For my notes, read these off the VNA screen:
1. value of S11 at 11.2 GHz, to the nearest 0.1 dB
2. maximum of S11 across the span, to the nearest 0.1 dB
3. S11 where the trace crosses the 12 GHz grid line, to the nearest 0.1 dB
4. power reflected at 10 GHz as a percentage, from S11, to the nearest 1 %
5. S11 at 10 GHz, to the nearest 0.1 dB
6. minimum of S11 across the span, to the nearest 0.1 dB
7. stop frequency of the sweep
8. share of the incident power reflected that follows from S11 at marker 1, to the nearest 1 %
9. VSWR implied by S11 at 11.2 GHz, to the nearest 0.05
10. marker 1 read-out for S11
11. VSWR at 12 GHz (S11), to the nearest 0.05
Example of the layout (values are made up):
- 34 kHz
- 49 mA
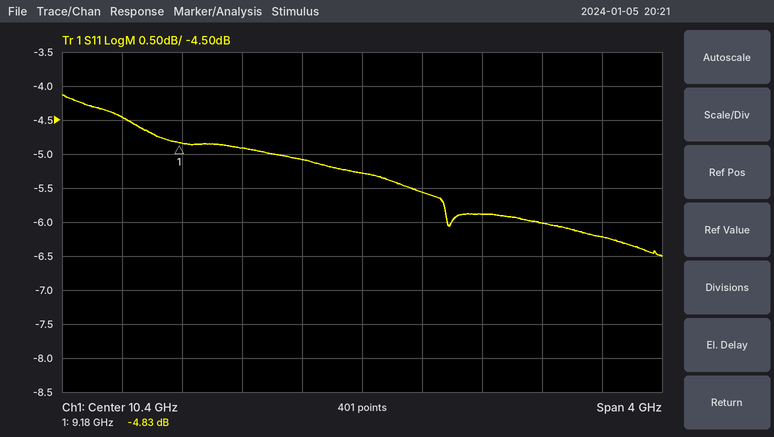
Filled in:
- -5.9 dB
- -4.1 dB
- -6.2 dB
- 31 %
- -5.1 dB
- -6.5 dB
- 12.4 GHz
- 33 %
- 3.05
- -4.83 dB
- 2.90
